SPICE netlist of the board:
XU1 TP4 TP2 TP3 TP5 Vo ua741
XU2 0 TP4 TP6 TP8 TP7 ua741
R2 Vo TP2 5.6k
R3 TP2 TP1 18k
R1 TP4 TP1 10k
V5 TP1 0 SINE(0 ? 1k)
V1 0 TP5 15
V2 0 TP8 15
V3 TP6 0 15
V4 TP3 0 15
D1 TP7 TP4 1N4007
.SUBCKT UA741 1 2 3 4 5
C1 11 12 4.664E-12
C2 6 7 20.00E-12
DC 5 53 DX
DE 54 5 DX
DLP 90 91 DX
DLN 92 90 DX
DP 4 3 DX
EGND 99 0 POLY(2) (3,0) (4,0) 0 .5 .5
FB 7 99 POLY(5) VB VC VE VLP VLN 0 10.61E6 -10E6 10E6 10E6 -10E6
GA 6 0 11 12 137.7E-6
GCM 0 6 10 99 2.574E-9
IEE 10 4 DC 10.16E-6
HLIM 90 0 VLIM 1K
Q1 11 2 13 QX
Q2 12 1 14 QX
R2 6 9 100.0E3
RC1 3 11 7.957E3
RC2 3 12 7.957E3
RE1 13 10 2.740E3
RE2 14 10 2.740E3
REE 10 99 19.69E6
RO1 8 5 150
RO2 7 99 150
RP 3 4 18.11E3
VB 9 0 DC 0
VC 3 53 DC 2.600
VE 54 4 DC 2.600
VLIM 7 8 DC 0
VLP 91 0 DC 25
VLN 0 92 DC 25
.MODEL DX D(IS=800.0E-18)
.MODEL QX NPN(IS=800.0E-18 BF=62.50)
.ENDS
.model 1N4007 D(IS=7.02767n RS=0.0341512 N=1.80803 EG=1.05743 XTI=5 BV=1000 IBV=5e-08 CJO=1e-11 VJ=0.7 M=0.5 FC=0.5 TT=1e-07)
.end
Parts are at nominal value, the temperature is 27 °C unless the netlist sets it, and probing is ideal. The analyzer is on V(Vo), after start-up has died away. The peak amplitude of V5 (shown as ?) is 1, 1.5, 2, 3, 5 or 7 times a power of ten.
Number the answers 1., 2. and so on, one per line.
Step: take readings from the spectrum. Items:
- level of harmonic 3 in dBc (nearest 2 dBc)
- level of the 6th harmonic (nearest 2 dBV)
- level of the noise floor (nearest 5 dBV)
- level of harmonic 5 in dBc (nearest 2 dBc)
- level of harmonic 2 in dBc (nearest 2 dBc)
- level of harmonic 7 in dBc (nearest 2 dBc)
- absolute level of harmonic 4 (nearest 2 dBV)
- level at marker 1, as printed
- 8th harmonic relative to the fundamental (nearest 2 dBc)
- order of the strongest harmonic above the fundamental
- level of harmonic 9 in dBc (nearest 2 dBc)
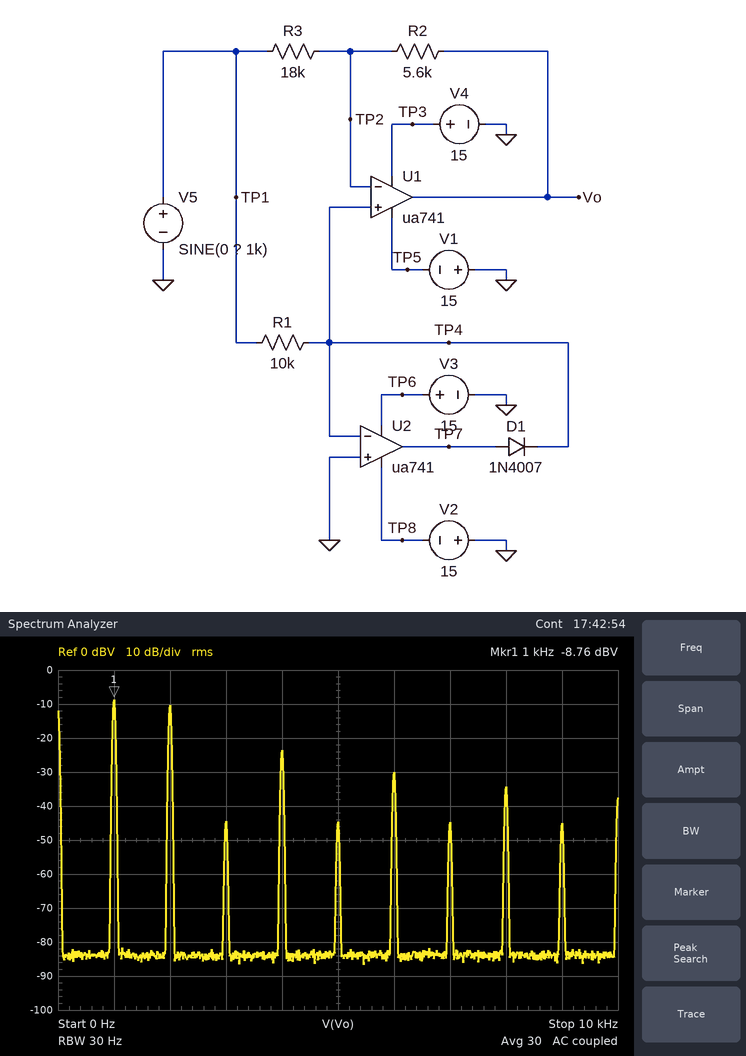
1. -36 dBc
2. -30 dBV
3. -85 dBV
4. -36 dBc
5. -2 dBc
6. -36 dBc
7. -24 dBV
8. -8.76 dBV
9. -26 dBc
10. 2
11. -36 dBc
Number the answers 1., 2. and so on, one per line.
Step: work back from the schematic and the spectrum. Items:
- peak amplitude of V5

1. 1.5 V
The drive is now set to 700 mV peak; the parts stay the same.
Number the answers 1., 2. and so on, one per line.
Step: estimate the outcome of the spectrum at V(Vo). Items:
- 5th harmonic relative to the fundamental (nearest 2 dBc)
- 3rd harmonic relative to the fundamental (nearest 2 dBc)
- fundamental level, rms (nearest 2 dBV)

1. -34 dBc
2. -34 dBc
3. -16 dBV
